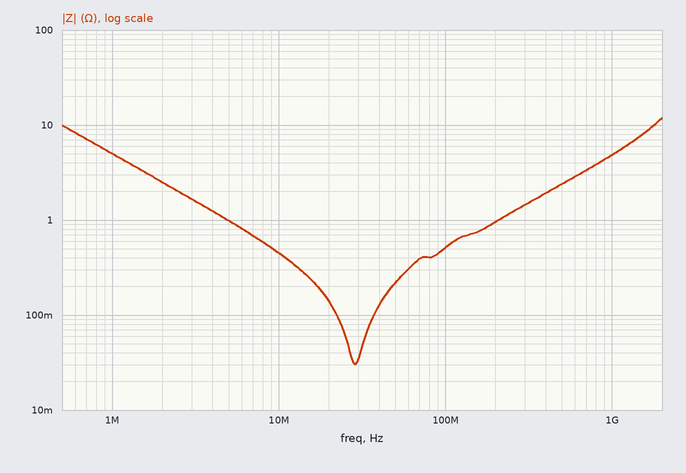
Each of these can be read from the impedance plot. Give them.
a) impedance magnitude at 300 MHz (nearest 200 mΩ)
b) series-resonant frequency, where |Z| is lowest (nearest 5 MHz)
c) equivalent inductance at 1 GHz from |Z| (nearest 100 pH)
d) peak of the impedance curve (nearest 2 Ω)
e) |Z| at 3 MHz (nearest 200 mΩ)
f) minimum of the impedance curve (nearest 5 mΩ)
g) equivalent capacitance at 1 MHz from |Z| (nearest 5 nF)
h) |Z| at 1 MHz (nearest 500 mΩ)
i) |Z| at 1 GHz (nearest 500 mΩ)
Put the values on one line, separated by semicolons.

1.4 Ω; 30 MHz; 800 pH; 12 Ω; 1.6 Ω; 30 mΩ; 30 nF; 5.0 Ω; 5.0 Ω
